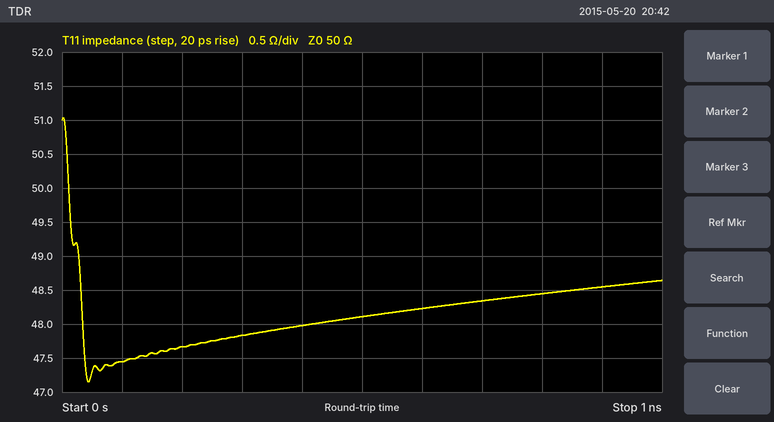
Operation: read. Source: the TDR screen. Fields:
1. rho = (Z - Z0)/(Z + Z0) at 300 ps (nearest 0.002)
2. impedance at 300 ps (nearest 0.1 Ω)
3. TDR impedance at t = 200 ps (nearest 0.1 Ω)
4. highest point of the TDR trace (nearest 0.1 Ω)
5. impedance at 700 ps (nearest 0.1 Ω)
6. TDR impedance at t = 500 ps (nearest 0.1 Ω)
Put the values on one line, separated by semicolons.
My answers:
-0.022; 47.8 Ω; 47.7 Ω; 51.0 Ω; 48.3 Ω; 48.1 Ω
